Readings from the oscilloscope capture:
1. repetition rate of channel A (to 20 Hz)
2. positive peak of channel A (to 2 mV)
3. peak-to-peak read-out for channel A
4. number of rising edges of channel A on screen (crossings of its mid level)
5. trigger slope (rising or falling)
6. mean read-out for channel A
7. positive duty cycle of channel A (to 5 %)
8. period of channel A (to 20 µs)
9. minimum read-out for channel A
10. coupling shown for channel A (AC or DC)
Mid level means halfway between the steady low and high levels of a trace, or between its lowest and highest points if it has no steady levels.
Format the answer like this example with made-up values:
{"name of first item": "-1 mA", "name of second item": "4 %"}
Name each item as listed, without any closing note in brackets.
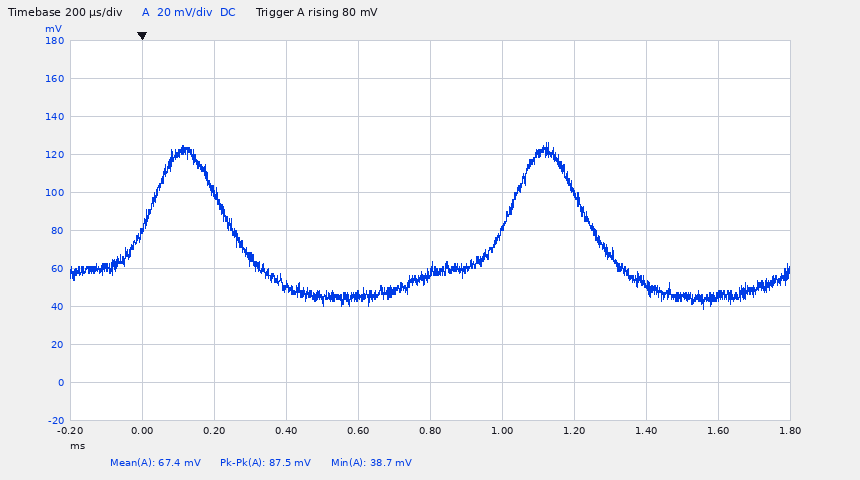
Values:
{"repetition rate of channel A": "1.00 kHz", "positive peak of channel A": "126 mV", "peak-to-peak read-out for channel A": "87.5 mV", "number of rising edges of channel A on screen": "2", "trigger slope": "rising", "mean read-out for channel A": "67.4 mV", "positive duty cycle of channel A": "25 %", "period of channel A": "1.00 ms", "minimum read-out for channel A": "38.7 mV", "coupling shown for channel A": "DC"}
